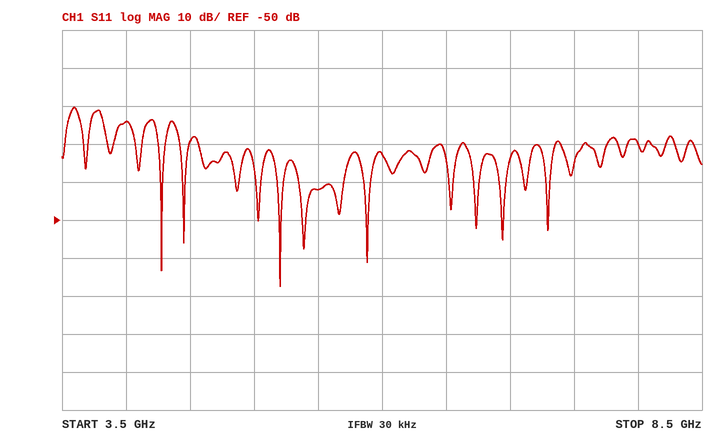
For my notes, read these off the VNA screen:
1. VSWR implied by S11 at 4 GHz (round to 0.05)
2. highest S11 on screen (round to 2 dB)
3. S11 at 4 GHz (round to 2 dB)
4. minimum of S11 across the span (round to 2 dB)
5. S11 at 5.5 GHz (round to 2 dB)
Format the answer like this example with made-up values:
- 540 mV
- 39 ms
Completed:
- 1.15
- -20 dB
- -24 dB
- -68 dB
- -42 dB
